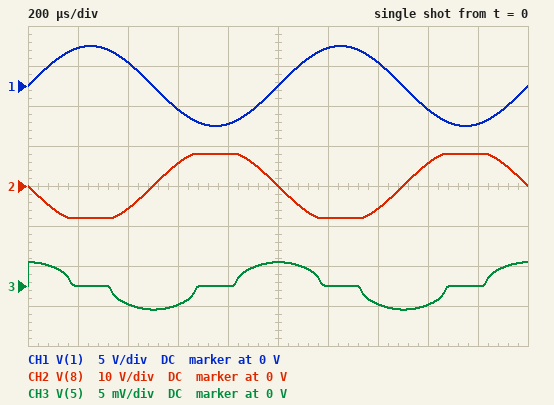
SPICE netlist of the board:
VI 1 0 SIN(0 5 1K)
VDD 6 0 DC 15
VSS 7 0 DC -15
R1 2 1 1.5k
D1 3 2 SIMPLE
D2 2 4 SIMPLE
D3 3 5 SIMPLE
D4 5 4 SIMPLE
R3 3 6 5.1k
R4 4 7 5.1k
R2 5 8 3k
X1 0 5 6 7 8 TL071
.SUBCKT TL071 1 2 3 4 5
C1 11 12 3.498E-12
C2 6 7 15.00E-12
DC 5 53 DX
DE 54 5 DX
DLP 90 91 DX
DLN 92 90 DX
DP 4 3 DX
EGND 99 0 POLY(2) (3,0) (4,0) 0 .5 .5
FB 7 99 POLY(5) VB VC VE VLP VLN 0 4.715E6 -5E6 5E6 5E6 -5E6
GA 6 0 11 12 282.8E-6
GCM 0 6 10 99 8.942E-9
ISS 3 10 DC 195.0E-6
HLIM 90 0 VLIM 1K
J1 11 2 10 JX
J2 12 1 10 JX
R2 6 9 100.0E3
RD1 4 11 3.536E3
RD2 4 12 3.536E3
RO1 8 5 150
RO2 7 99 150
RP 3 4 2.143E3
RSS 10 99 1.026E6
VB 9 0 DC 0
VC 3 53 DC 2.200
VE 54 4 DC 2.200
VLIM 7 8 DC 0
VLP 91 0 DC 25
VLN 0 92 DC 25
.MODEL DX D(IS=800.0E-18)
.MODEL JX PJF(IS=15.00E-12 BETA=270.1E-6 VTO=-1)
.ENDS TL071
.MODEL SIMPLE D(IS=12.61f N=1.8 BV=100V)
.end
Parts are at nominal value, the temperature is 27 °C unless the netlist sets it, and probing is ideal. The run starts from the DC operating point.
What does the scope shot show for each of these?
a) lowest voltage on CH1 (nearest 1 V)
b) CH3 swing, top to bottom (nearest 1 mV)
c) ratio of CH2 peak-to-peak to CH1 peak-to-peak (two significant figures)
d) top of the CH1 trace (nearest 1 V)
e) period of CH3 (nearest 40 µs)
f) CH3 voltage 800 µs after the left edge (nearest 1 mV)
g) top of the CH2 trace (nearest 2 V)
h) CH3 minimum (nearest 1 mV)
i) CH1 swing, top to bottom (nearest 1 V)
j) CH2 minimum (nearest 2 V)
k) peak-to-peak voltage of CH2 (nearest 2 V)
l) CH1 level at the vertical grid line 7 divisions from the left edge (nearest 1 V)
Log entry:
-5 V
6 mV
1.6
5 V
1.00 ms
0 V
8 V
-3 mV
10 V
-8 V
16 V
3 V
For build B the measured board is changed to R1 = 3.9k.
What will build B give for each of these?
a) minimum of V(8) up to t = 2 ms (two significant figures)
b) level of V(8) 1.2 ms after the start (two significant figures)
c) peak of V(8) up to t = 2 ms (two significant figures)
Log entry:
-3.8 V
-3.6 V
3.8 V
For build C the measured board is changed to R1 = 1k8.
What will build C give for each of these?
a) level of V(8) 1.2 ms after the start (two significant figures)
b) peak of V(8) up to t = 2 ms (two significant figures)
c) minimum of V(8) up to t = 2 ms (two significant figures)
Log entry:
-7.6 V
7.9 V
-7.9 V
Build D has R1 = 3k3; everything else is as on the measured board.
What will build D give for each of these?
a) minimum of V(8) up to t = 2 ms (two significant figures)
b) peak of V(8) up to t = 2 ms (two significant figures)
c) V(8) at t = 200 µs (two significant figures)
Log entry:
-4.5 V
4.5 V
-4.2 V
